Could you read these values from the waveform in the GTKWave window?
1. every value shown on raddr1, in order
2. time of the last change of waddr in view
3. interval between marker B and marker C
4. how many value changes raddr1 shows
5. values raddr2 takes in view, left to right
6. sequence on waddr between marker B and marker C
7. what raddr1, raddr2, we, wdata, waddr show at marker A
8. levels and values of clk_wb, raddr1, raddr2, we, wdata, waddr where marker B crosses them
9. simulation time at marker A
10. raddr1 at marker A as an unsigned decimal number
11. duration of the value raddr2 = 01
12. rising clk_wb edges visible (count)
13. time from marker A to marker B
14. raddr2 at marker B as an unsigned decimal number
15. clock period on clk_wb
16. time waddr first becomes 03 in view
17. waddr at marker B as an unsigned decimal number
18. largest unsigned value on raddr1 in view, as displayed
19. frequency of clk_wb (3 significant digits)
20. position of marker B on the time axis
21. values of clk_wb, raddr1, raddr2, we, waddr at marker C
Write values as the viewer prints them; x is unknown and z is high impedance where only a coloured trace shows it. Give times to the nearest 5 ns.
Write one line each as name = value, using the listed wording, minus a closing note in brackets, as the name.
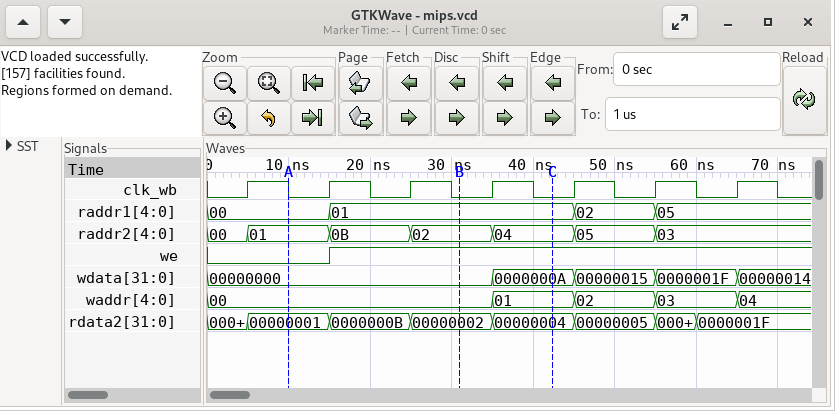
every value shown on raddr1, in order = 00, 01, 02, 05
time of the last change of waddr in view = 65 ns
interval between marker B and marker C = 10 ns
how many value changes raddr1 shows = 3
values raddr2 takes in view, left to right = 00, 01, 0B, 02, 04, 05, 03
sequence on waddr between marker B and marker C = 00, 01
what raddr1, raddr2, we, wdata, waddr show at marker A = raddr1=00, raddr2=01, we=0, wdata=00000000, waddr=00
levels and values of clk_wb, raddr1, raddr2, we, wdata, waddr where marker B crosses them = clk_wb=0, raddr1=01, raddr2=02, we=1, wdata=00000000, waddr=00
simulation time at marker A = 10 ns
raddr1 at marker A as an unsigned decimal number = 0
duration of the value raddr2 = 01 = 10 ns
rising clk_wb edges visible = 7
time from marker A to marker B = 20 ns
raddr2 at marker B as an unsigned decimal number = 2
clock period on clk_wb = 10 ns
time waddr first becomes 03 in view = 55 ns
waddr at marker B as an unsigned decimal number = 0
largest unsigned value on raddr1 in view, as displayed = 05
frequency of clk_wb = 100 MHz
position of marker B on the time axis = 30 ns
values of clk_wb, raddr1, raddr2, we, waddr at marker C = clk_wb=0, raddr1=01, raddr2=04, we=1, waddr=01
